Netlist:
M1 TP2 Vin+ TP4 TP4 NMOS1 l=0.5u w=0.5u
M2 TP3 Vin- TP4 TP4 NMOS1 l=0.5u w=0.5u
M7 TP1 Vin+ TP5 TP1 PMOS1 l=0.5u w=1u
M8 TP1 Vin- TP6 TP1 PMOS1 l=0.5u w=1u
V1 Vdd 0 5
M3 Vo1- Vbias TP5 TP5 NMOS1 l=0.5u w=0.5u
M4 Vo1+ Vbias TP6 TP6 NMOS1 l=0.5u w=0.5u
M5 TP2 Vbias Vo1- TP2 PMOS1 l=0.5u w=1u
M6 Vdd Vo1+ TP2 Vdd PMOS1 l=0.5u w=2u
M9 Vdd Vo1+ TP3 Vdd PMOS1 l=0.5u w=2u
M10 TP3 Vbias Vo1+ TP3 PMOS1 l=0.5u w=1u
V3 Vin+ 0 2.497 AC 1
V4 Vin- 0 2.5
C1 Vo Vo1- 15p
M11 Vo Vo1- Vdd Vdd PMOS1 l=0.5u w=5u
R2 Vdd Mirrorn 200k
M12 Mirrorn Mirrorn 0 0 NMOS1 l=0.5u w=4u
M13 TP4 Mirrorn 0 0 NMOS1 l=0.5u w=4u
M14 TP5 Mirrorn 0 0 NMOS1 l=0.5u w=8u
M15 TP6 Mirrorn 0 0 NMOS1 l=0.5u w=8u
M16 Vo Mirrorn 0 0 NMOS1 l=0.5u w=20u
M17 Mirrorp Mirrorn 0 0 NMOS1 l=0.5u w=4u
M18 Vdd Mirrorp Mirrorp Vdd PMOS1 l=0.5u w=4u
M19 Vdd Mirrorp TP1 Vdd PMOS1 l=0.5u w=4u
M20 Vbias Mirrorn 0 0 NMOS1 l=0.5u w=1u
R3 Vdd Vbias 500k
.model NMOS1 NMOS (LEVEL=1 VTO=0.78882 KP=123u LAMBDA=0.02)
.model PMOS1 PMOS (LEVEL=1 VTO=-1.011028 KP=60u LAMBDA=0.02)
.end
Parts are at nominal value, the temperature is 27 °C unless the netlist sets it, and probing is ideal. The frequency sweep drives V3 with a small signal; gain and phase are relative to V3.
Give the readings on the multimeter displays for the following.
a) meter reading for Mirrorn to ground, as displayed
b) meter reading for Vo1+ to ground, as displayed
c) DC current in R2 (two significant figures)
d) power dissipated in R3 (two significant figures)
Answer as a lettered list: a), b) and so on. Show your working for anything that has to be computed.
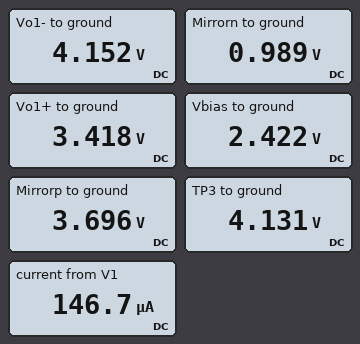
a) 0.989 V
b) 3.418 V
c) (5 V - 989 mV) / 200 kΩ = 20 µA
d) (5 V - 2.422 V)^2 / 500 kΩ = 13 µW
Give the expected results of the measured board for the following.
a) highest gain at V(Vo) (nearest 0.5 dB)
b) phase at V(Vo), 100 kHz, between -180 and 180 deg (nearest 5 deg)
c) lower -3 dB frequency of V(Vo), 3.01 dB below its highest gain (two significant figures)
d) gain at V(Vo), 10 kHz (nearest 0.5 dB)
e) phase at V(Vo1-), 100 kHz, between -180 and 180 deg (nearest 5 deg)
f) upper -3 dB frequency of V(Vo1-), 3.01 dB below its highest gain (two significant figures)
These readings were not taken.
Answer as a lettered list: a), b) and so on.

a) -20.0 dB
b) -170 deg
c) 20 kHz
d) -27.0 dB
e) 100 deg
f) 20 kHz
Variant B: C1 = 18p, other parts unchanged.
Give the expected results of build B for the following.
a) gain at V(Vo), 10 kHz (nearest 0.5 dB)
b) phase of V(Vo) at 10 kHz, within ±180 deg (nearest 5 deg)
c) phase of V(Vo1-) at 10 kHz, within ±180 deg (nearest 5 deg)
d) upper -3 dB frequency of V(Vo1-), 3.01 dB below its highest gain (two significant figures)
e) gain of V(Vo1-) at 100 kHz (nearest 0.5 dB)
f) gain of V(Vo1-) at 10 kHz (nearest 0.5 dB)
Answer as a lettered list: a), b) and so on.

a) -25.5 dB
b) -120 deg
c) 150 deg
d) 17 kHz
e) 19.0 dB
f) 33.0 dB
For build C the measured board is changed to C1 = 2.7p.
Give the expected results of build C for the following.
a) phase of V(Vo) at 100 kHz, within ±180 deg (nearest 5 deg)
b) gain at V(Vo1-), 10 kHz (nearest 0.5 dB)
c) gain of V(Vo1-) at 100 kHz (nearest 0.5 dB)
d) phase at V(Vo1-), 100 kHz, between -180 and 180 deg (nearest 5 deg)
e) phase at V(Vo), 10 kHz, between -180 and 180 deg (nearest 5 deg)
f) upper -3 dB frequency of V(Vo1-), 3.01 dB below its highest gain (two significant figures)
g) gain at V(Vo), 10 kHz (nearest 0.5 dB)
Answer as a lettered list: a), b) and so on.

a) -130 deg
b) 34.5 dB
c) 32.0 dB
d) 140 deg
e) -95 deg
f) 110 kHz
g) -41.0 dB
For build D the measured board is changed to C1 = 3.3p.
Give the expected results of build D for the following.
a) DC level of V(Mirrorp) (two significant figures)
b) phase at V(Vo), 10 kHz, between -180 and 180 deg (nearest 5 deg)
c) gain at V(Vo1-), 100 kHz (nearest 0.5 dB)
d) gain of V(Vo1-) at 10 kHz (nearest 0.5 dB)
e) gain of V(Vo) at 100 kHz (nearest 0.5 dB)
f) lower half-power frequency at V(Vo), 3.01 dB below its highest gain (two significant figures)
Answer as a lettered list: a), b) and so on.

a) 3.7 V
b) -95 deg
c) 31.0 dB
d) 34.5 dB
e) -22.5 dB
f) 92 kHz
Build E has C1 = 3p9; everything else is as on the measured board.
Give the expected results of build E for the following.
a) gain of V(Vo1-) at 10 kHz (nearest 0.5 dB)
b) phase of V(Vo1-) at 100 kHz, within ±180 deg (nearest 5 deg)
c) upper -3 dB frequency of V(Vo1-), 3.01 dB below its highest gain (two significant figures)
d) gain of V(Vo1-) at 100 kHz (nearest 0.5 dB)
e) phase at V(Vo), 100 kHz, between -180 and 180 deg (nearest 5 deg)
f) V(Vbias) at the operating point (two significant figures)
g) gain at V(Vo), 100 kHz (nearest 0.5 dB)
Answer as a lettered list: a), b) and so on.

a) 34.5 dB
b) 130 deg
c) 78 kHz
d) 30.0 dB
e) -140 deg
f) 2.4 V
g) -22.0 dB
